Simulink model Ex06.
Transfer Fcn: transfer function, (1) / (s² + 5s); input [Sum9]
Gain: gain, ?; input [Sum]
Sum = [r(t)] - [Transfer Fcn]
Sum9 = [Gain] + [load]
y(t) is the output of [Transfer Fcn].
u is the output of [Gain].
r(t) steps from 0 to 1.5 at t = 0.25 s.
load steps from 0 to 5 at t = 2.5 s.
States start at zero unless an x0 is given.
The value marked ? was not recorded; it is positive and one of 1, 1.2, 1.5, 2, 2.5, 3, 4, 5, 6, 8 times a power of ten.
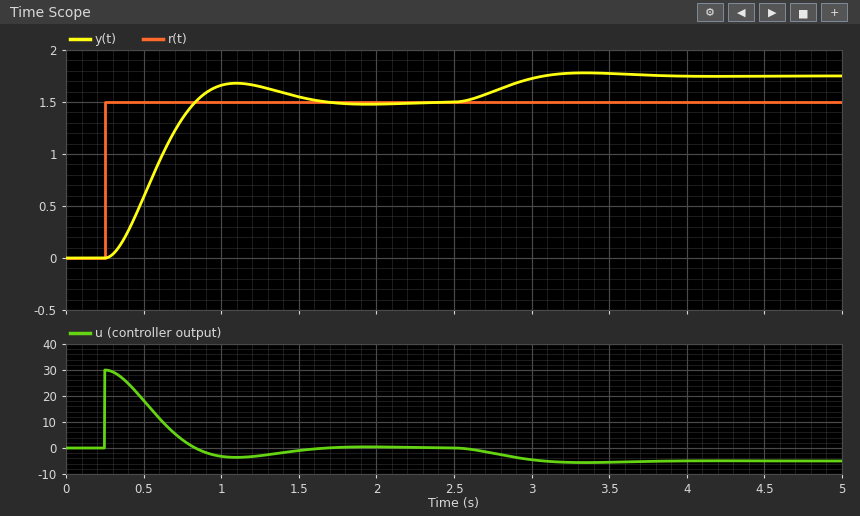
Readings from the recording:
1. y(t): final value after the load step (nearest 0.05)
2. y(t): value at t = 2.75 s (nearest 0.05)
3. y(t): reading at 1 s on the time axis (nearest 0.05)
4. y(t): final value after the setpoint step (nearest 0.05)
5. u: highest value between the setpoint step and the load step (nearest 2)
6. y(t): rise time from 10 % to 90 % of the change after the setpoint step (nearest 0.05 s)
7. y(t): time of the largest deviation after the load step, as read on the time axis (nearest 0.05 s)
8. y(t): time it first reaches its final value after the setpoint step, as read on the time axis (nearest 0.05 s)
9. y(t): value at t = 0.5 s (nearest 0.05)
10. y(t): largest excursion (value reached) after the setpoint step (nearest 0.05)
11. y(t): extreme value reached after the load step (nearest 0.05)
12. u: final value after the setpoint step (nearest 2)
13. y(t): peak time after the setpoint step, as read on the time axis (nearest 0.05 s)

1.75
1.60
1.65
1.50
30
0.40 s
3.35 s
0.85 s
0.60
1.70
1.80
0
1.10 s
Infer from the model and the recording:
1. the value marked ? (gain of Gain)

20
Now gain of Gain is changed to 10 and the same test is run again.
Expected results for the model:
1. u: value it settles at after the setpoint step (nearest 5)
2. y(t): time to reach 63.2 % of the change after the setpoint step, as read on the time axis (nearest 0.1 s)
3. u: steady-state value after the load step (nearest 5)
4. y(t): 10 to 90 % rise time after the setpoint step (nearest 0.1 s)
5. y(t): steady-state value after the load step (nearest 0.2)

0
0.8 s
-5
0.8 s
2.0
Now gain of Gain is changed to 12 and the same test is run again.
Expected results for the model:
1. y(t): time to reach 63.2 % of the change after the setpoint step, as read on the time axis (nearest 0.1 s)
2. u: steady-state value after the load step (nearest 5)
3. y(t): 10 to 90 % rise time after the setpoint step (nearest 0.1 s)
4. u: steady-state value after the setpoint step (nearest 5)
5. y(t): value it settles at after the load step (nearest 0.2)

0.8 s
-5
0.6 s
0
2.0
